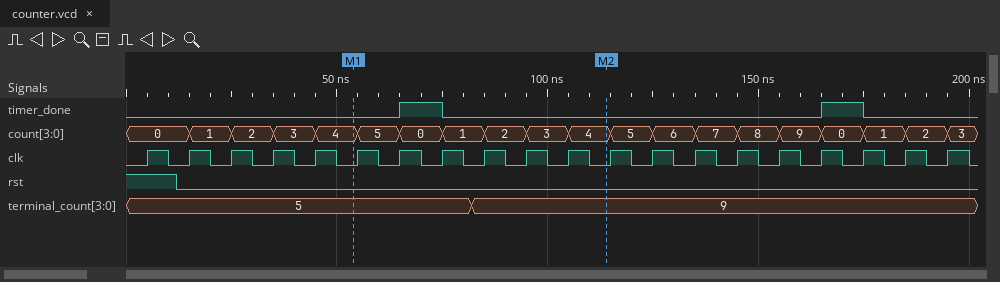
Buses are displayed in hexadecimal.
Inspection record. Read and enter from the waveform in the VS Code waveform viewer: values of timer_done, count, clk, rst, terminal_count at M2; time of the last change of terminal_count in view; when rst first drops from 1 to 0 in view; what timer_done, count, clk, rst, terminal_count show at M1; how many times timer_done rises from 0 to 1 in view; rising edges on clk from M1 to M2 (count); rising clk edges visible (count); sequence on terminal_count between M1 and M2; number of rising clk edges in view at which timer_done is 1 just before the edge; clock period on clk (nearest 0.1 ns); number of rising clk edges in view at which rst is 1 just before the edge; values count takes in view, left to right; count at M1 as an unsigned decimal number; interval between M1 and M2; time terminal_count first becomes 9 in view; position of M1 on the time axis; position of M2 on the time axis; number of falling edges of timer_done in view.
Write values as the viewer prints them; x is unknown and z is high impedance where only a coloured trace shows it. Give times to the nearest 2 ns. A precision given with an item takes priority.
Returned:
timer_done=0, count=4, clk=0, rst=0, terminal_count=9
82 ns
12 ns
timer_done=0, count=4, clk=0, rst=0, terminal_count=5
2
6
20
5, 9
2
10 ns
1
0, 1, 2, 3, 4, 5, 0, 1, 2, 3, 4, 5, 6, 7, 8, 9, 0, 1, 2, 3
4
60 ns
82 ns
54 ns
114 ns
2
